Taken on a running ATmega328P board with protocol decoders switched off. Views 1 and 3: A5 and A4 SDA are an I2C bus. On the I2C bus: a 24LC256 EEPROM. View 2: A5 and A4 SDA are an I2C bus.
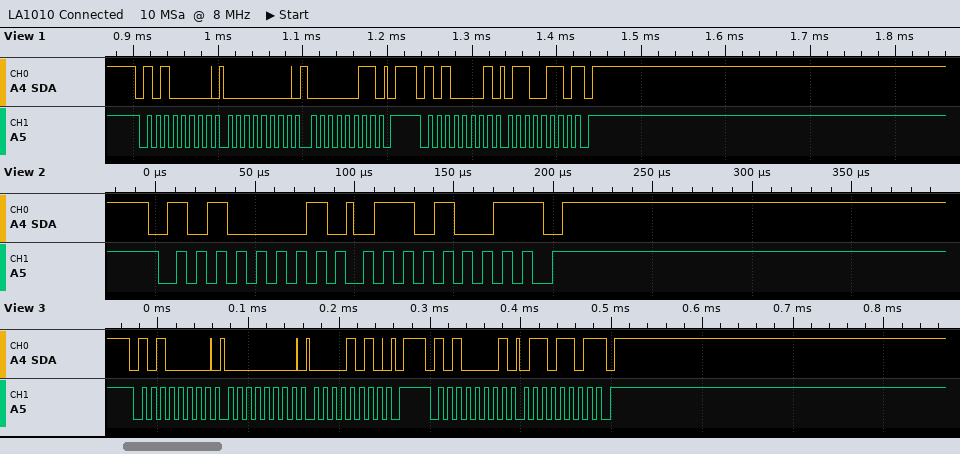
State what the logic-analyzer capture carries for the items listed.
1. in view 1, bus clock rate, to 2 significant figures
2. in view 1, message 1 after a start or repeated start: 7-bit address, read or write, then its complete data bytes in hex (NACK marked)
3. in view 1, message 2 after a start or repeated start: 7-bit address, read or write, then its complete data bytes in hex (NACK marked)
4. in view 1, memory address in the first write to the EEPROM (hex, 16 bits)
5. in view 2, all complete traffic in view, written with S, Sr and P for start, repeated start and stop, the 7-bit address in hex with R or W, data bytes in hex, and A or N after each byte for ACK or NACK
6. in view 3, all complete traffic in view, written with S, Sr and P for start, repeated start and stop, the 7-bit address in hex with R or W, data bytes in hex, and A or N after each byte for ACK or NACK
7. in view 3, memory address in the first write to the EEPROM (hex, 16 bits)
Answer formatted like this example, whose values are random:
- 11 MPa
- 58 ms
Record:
- 100 kHz
- 0x50 write: 00 03
- 0x50 read: 66 NACK
- 0x0003
- S 50R A 69 N P
- S 50W A 00 A 0A A P S 50R A 6D N P
- 0x000A
